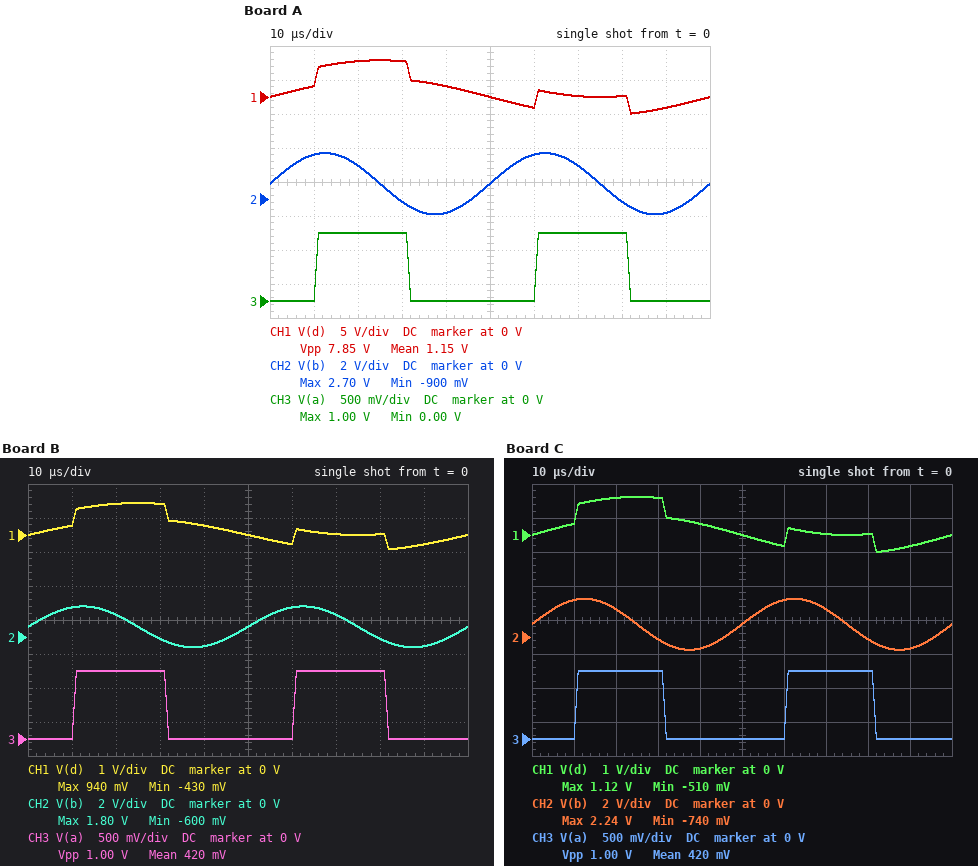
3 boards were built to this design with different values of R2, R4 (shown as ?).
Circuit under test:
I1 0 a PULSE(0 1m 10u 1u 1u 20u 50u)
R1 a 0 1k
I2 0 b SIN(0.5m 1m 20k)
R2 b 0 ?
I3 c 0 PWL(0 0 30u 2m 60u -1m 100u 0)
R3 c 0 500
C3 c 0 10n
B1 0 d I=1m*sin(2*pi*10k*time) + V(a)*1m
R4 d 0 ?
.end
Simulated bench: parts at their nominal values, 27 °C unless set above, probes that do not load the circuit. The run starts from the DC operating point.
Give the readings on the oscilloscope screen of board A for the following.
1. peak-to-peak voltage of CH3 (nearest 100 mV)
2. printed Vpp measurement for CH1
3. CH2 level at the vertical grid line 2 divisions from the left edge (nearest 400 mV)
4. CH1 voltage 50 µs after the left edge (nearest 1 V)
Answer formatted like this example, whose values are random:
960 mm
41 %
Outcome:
1.0 V
7.85 V
2.0 V
0 V
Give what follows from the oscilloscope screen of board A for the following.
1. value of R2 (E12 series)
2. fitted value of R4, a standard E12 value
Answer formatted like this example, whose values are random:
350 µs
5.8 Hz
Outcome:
1.8 kΩ
2.7 kΩ
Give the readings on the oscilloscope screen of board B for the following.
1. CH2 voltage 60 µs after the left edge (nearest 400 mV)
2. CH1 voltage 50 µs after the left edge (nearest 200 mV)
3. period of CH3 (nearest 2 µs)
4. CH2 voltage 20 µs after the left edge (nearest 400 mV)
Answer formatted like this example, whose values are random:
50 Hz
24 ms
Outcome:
1.6 V
0 V
50 µs
1.2 V
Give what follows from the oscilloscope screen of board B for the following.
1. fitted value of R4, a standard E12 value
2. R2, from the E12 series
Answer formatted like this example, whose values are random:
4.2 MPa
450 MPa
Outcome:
470 Ω
1.2 kΩ
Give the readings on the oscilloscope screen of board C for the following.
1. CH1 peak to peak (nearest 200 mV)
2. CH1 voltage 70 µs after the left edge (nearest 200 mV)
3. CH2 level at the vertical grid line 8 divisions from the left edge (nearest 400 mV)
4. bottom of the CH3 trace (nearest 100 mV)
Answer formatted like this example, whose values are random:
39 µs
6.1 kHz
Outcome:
1.6 V
0 V
0 V
0 V
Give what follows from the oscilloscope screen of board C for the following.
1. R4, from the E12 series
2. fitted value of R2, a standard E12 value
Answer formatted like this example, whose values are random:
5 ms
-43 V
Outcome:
560 Ω
1.5 kΩ
